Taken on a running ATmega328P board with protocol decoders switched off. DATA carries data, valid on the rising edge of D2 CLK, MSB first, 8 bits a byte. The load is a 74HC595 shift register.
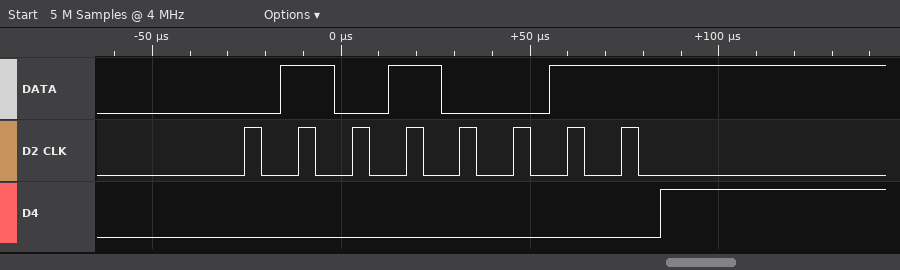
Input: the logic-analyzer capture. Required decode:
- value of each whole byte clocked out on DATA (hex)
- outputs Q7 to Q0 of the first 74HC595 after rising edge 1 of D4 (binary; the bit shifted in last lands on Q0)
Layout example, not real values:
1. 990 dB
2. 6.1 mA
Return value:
1. 0x53
2. 01010011
